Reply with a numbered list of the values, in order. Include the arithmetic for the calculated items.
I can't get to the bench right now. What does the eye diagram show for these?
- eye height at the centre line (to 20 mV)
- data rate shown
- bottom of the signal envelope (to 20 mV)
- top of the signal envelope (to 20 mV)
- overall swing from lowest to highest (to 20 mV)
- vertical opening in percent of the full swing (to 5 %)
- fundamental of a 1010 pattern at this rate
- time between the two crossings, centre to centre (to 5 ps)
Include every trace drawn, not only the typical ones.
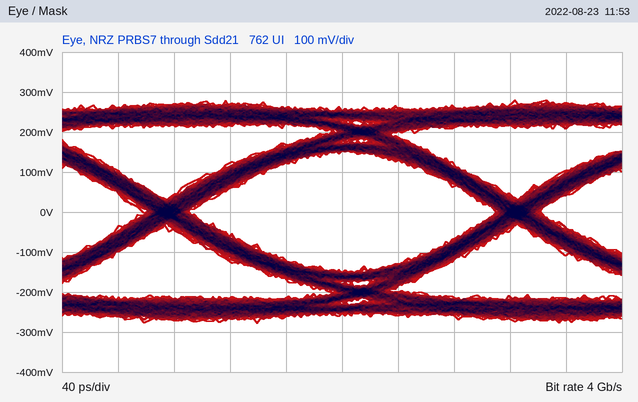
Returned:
1. 300 mV
2. 4 Gb/s
3. -280 mV
4. 280 mV
5. 560 mV
6. 300 mV / 560 mV ≈ 53.6 %, so 55 % to the nearest 5 %
7. 2 GHz
8. 250 ps
